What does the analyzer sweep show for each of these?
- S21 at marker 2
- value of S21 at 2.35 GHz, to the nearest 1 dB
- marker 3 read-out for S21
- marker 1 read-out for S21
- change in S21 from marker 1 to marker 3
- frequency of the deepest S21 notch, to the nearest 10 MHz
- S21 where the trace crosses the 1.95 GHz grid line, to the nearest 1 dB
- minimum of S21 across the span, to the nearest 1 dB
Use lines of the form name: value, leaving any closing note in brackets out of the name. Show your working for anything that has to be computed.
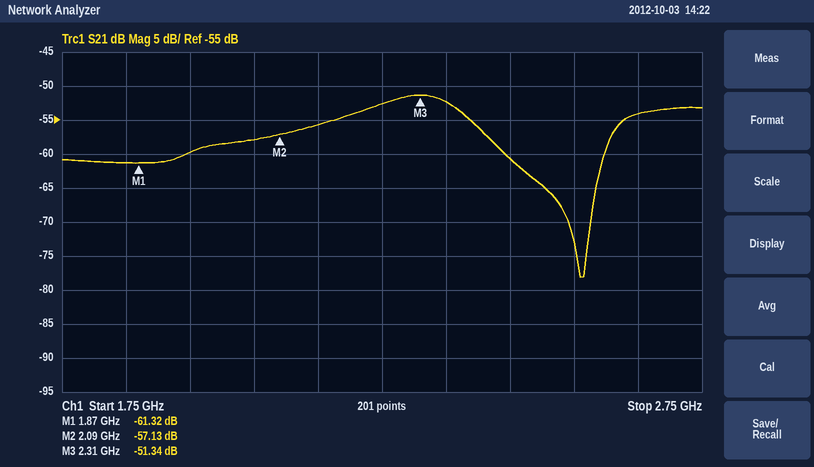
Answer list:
S21 at marker 2: -57.13 dB
value of S21 at 2.35 GHz, to the nearest 1 dB: -52 dB
marker 3 read-out for S21: -51.34 dB
marker 1 read-out for S21: -61.32 dB
change in S21 from marker 1 to marker 3: -51.34 − (-61.32) = 9.98 dB
frequency of the deepest S21 notch, to the nearest 10 MHz: 2.56 GHz
S21 where the trace crosses the 1.95 GHz grid line, to the nearest 1 dB: -60 dB
minimum of S21 across the span, to the nearest 1 dB: -78 dB
